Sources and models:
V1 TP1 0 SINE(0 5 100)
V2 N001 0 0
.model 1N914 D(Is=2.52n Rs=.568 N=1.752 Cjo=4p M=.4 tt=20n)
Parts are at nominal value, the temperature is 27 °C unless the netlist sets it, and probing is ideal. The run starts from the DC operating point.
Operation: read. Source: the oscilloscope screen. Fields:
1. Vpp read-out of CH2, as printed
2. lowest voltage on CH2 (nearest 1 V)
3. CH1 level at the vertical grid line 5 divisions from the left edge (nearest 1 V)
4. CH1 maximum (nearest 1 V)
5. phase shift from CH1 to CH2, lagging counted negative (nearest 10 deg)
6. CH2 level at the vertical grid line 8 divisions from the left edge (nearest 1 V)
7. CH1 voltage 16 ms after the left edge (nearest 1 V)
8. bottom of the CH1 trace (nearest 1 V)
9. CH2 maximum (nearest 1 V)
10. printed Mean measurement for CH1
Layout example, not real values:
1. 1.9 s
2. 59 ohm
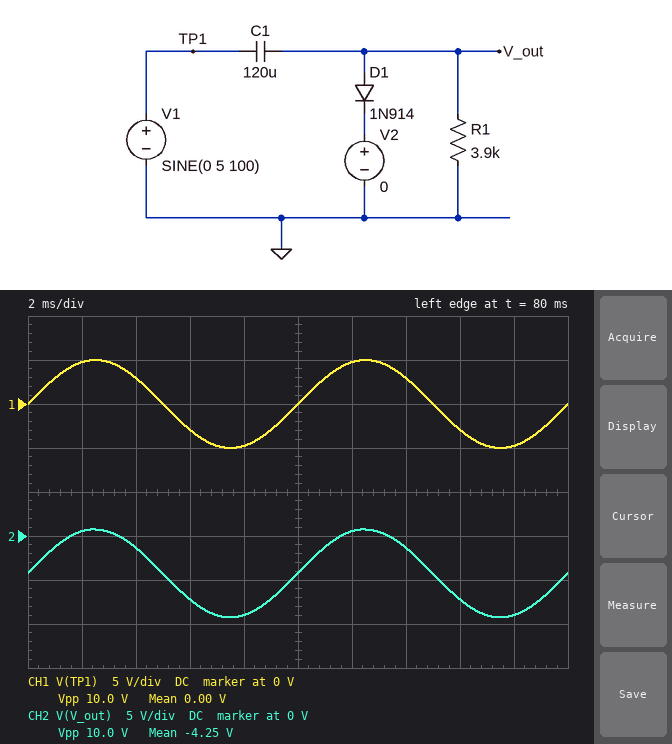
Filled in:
1. 10.0 V
2. -9 V
3. 0 V
4. 5 V
5. 0 deg
6. -7 V
7. -3 V
8. -5 V
9. 1 V
10. 0.00 V
